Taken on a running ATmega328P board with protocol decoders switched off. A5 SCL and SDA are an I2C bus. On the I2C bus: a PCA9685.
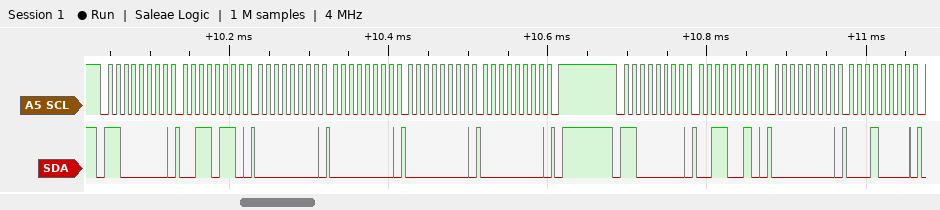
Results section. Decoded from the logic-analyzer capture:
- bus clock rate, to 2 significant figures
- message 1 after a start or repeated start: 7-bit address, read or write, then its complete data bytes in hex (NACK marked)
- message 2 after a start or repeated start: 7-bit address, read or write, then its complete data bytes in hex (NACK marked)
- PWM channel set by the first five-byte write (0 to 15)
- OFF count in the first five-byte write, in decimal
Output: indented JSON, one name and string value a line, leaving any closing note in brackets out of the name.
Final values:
{
  "bus clock rate, to 2 significant figures": "100 kHz",
  "message 1 after a start or repeated start: 7-bit address, read or write, then its complete data bytes in hex": "0x60 write: 36 00 00 00 00",
  "message 2 after a start or repeated start: 7-bit address, read or write, then its complete data bytes in hex": "0x60 write: 32 00 10",
  "PWM channel set by the first five-byte write": "12",
  "OFF count in the first five-byte write, in decimal": "0"
}
